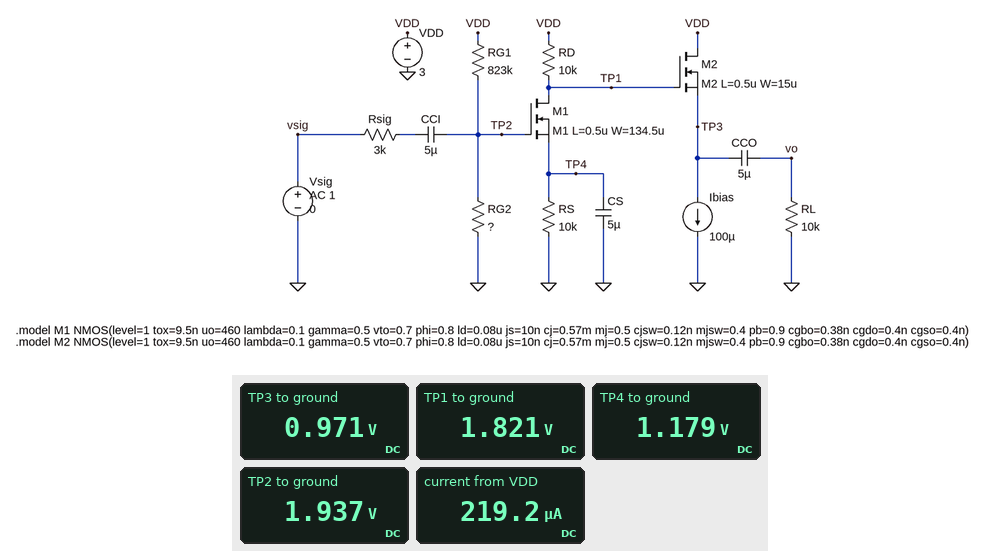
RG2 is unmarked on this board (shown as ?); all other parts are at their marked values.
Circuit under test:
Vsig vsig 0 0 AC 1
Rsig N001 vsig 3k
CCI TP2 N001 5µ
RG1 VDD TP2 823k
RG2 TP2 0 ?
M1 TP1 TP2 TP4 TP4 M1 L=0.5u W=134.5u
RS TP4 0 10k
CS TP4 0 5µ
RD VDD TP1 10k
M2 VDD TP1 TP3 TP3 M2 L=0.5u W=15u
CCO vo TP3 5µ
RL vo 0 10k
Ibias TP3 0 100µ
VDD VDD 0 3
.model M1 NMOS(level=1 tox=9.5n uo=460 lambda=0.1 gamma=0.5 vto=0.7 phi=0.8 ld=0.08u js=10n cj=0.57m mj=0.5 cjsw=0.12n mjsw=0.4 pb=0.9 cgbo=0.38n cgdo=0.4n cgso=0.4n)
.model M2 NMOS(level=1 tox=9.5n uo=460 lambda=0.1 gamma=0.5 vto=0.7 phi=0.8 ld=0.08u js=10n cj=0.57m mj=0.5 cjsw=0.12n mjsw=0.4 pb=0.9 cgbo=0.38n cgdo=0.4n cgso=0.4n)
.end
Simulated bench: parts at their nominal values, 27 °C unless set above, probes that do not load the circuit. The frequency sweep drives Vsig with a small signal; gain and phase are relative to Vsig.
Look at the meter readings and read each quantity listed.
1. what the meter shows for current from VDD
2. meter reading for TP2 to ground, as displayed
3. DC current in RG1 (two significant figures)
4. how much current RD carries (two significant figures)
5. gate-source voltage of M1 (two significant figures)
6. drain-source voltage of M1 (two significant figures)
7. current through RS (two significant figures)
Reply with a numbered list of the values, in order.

1. 219.2 µA
2. 1.937 V
3. 1.3 µA
4. 120 µA
5. 760 mV
6. 640 mV
7. 120 µA
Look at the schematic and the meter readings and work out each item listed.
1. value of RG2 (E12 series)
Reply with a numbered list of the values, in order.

1. 1.5 MΩ
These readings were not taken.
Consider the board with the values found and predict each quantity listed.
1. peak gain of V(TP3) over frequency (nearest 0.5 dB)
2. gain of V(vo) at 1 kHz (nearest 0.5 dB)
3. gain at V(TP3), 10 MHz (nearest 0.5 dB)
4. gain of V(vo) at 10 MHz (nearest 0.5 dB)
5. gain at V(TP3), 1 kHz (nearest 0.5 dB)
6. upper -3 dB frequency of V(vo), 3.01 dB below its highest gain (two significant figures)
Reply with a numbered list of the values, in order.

1. 30.5 dB
2. 30.5 dB
3. 30.0 dB
4. 30.0 dB
5. 30.5 dB
6. 23 MHz
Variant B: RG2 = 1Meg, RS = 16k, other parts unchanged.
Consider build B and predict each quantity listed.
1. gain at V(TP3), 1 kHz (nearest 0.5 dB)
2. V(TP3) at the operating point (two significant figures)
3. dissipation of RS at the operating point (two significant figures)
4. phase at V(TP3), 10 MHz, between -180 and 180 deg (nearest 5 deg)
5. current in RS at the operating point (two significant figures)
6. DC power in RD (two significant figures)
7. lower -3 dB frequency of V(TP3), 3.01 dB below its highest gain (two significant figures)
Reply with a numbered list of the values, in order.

1. 28.0 dB
2. 1.6 V
3. 51 µW
4. 160 deg
5. 57 µA
6. 32 µW
7. 91 Hz
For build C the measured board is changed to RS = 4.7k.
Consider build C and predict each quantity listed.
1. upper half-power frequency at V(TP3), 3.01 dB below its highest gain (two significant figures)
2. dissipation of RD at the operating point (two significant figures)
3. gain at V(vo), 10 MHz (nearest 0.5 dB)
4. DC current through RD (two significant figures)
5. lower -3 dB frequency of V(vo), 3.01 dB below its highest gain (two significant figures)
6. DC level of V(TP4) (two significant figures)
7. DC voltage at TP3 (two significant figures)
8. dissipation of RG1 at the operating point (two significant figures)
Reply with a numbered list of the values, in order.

1. 200 MHz
2. 410 µW
3. -28.5 dB
4. 200 µA
5. 6.4 Hz
6. 960 mV
7. 120 mV
8. 1.4 µW
